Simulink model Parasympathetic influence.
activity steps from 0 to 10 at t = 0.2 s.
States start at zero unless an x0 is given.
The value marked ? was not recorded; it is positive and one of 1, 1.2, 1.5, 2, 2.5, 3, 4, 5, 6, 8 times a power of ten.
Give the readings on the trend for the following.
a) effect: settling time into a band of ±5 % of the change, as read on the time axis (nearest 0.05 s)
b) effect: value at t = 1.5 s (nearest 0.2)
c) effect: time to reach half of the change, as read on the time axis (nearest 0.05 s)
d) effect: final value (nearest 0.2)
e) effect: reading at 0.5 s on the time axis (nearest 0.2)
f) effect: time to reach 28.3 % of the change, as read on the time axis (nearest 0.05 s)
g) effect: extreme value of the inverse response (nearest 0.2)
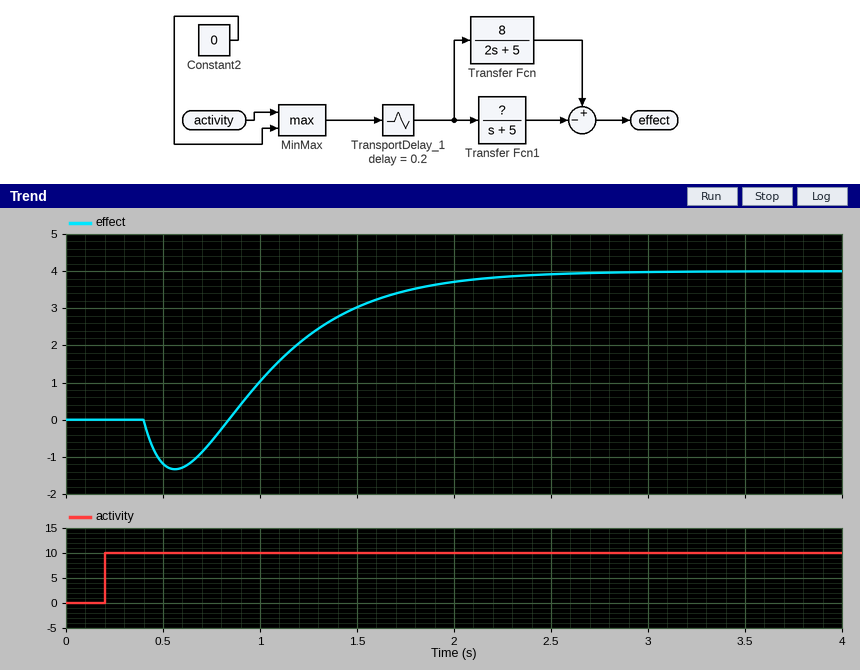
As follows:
2.15 s
3.0
1.20 s
4.0
-1.2
1.00 s
-1.4
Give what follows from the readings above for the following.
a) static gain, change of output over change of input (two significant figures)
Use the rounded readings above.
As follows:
0.40
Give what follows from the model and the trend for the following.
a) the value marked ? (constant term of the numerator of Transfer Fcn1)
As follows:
6
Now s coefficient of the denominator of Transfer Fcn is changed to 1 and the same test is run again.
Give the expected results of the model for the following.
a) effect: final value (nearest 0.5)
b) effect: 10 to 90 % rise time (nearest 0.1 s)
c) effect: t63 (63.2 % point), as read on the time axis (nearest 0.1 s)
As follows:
4.0
0.4 s
0.6 s
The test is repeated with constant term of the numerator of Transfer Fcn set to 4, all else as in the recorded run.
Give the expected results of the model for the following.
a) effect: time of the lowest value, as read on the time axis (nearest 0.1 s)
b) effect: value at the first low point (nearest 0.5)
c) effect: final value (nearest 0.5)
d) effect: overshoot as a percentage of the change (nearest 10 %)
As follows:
0.8 s
-5.5
-4.0
30 %
